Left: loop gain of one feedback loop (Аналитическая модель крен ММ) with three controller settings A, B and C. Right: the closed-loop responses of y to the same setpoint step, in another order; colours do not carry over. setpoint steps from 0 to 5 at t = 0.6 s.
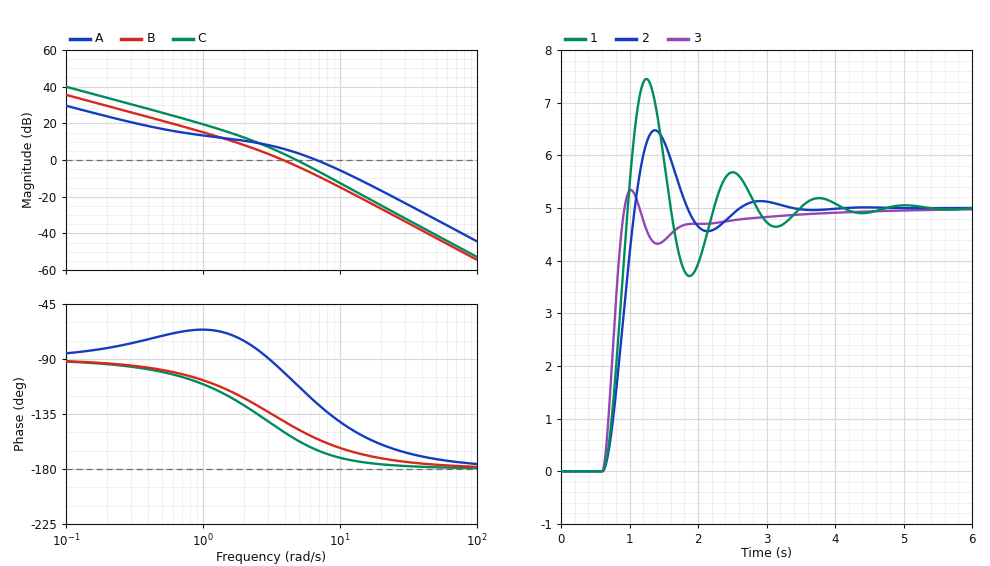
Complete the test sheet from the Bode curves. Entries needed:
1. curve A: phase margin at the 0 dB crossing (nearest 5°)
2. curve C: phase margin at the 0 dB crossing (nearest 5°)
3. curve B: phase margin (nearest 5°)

55°
25°
40°
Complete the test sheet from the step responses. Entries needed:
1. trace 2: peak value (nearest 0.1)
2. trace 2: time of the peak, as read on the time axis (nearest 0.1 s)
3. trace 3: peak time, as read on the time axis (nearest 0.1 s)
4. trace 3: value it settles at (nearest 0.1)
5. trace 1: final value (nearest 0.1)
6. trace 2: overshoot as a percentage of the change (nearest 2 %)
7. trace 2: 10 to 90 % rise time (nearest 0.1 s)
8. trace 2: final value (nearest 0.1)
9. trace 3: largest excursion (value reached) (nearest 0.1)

6.5
1.4 s
1.0 s
5.0
5.0
30 %
0.3 s
5.0
5.3
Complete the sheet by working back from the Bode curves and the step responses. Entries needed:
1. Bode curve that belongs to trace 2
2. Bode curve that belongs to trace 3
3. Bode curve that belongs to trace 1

B
A
C
